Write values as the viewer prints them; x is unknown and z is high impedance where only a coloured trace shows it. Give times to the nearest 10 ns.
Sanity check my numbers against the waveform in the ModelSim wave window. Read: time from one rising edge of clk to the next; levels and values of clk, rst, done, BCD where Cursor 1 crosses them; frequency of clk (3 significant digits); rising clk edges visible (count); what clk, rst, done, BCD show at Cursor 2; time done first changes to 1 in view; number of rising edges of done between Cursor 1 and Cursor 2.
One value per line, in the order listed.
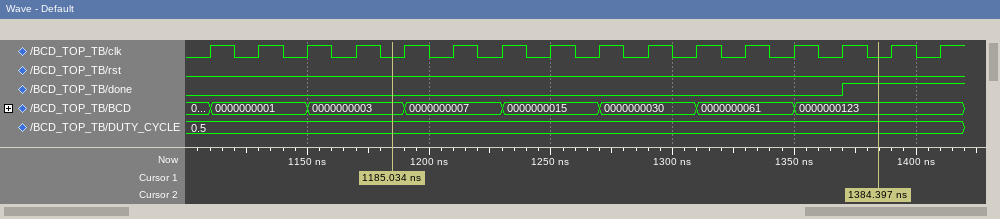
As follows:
20 ns
clk=0, rst=0, done=0, BCD=0000000003
50.0 MHz
16
clk=0, rst=0, done=1, BCD=0000000123
1370 ns
1
